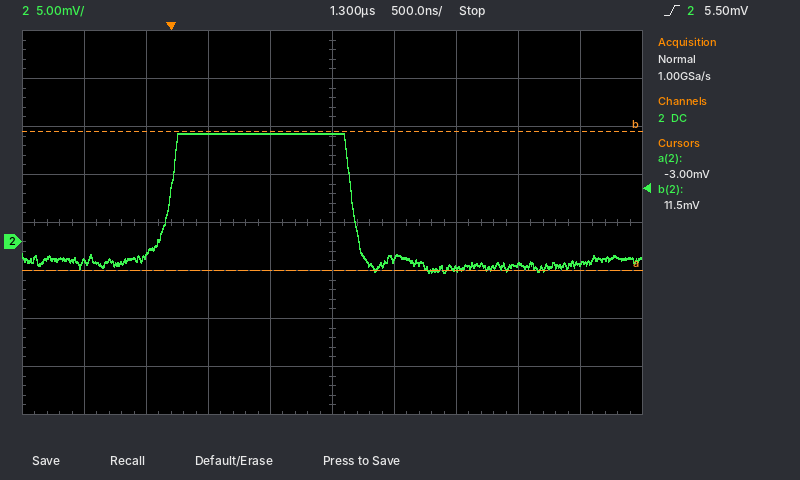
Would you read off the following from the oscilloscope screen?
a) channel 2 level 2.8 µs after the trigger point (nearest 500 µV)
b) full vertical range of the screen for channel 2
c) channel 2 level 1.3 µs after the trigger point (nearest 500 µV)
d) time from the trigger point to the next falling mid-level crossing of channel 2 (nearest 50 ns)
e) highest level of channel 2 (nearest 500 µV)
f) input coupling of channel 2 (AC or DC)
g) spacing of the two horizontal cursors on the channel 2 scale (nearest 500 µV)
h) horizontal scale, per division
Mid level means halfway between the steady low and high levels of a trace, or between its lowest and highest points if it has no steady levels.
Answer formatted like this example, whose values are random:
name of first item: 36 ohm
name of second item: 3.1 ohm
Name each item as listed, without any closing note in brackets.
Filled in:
channel 2 level 2.8 µs after the trigger point: -2.5 mV
full vertical range of the screen for channel 2: 40 mV
channel 2 level 1.3 µs after the trigger point: 11.5 mV
time from the trigger point to the next falling mid-level crossing of channel 2: 1.45 µs
highest level of channel 2: 11.5 mV
input coupling of channel 2: DC
spacing of the two horizontal cursors on the channel 2 scale: 14.5 mV
horizontal scale, per division: 500 ns
